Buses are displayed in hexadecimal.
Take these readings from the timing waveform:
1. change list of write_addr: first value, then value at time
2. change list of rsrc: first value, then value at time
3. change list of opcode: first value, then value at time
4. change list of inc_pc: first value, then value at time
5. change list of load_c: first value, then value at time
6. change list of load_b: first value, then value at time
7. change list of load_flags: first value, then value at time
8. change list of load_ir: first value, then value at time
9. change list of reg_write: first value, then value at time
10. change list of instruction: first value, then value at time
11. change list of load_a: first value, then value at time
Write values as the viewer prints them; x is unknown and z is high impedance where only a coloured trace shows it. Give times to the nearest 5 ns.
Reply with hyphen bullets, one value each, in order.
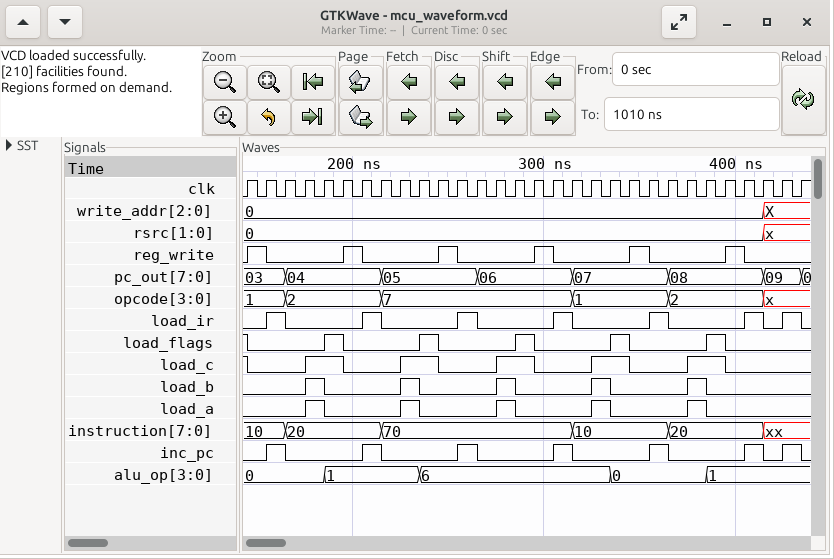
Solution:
- 0, X at 415 ns
- 0, x at 415 ns
- 1, 2 at 165 ns, 7 at 215 ns, 1 at 315 ns, 2 at 365 ns, x at 415 ns
- 0, 1 at 155 ns, 0 at 165 ns, 1 at 205 ns, 0 at 215 ns, 1 at 255 ns, 0 at 265 ns, 1 at 305 ns, 0 at 315 ns, 1 at 355 ns, 0 at 365 ns, 1 at 405 ns, 0 at 415 ns, 1 at 425 ns, 0 at 435 ns
- 1, 0 at 145 ns, 1 at 175 ns, 0 at 195 ns, 1 at 225 ns, 0 at 245 ns, 1 at 275 ns, 0 at 295 ns, 1 at 325 ns, 0 at 345 ns, 1 at 375 ns, 0 at 395 ns
- 0, 1 at 175 ns, 0 at 185 ns, 1 at 225 ns, 0 at 235 ns, 1 at 275 ns, 0 at 285 ns, 1 at 325 ns, 0 at 335 ns, 1 at 375 ns, 0 at 385 ns
- 1, 0 at 145 ns, 1 at 185 ns, 0 at 195 ns, 1 at 235 ns, 0 at 245 ns, 1 at 285 ns, 0 at 295 ns, 1 at 335 ns, 0 at 345 ns, 1 at 385 ns, 0 at 395 ns
- 0, 1 at 155 ns, 0 at 165 ns, 1 at 205 ns, 0 at 215 ns, 1 at 255 ns, 0 at 265 ns, 1 at 305 ns, 0 at 315 ns, 1 at 355 ns, 0 at 365 ns, 1 at 405 ns, 0 at 415 ns, 1 at 425 ns, 0 at 435 ns
- 0, 1 at 145 ns, 0 at 155 ns, 1 at 195 ns, 0 at 205 ns, 1 at 245 ns, 0 at 255 ns, 1 at 295 ns, 0 at 305 ns, 1 at 345 ns, 0 at 355 ns, 1 at 395 ns, 0 at 405 ns
- 10, 20 at 165 ns, 70 at 215 ns, 10 at 315 ns, 20 at 365 ns, xx at 415 ns
- 0, 1 at 175 ns, 0 at 185 ns, 1 at 225 ns, 0 at 235 ns, 1 at 275 ns, 0 at 285 ns, 1 at 325 ns, 0 at 335 ns, 1 at 375 ns, 0 at 385 ns
